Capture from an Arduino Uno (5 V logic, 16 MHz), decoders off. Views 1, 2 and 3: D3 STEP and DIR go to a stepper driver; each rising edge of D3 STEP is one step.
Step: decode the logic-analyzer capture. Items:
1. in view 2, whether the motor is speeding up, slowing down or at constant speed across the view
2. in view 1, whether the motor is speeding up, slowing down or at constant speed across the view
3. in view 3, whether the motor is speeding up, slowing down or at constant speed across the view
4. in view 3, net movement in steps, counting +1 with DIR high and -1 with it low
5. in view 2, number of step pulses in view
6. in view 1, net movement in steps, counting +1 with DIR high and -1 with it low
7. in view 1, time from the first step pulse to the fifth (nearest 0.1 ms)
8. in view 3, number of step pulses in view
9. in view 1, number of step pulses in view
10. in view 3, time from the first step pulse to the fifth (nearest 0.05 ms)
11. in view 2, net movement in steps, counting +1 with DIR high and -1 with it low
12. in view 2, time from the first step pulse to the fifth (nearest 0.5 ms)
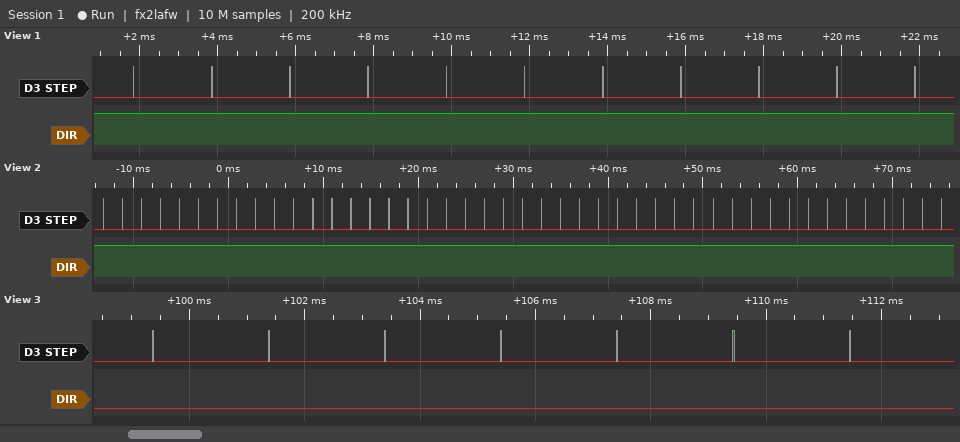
constant speed
constant speed
constant speed
-7
45
+11
8.0 ms
7
11
8.05 ms
+45
8.0 ms
